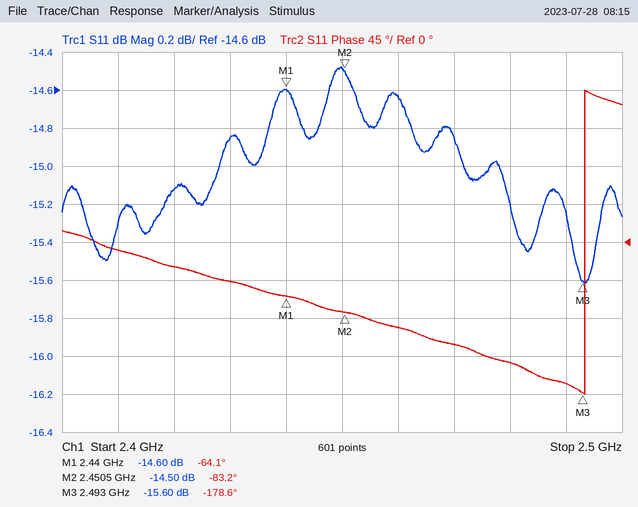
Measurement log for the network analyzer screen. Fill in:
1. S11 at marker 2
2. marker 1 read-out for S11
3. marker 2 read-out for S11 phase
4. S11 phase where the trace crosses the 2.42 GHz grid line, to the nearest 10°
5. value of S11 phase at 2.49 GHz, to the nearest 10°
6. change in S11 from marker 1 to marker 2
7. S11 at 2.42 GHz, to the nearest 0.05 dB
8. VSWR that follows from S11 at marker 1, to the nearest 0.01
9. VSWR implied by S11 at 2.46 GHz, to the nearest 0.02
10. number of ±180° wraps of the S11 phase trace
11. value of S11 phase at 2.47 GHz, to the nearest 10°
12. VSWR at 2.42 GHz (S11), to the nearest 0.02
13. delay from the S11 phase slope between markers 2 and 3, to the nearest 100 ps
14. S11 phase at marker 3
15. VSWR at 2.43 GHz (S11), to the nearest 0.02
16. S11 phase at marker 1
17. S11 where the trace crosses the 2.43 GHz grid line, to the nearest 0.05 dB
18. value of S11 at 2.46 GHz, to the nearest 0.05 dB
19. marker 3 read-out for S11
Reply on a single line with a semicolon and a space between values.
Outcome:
-14.50 dB; -14.60 dB; -83.2°; -30°; -170°; 0.10 dB; -15.10 dB; 1.46; 1.46; 1; -120°; 1.42; 6.2 ns; -178.6°; 1.44; -64.1°; -14.85 dB; -14.65 dB; -15.60 dB
